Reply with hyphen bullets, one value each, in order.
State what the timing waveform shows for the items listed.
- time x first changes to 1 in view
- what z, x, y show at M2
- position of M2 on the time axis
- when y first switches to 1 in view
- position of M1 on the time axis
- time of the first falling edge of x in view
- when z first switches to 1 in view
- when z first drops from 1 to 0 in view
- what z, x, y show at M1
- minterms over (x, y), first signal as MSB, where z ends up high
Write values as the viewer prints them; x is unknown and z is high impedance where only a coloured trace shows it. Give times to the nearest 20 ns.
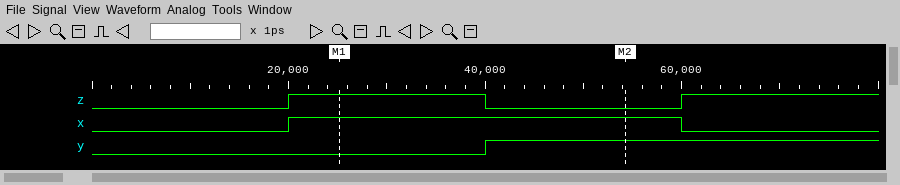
- 20 ns
- z=0, x=1, y=1
- 60 ns
- 40 ns
- 20 ns
- 60 ns
- 20 ns
- 40 ns
- z=1, x=1, y=0
- 1, 2
